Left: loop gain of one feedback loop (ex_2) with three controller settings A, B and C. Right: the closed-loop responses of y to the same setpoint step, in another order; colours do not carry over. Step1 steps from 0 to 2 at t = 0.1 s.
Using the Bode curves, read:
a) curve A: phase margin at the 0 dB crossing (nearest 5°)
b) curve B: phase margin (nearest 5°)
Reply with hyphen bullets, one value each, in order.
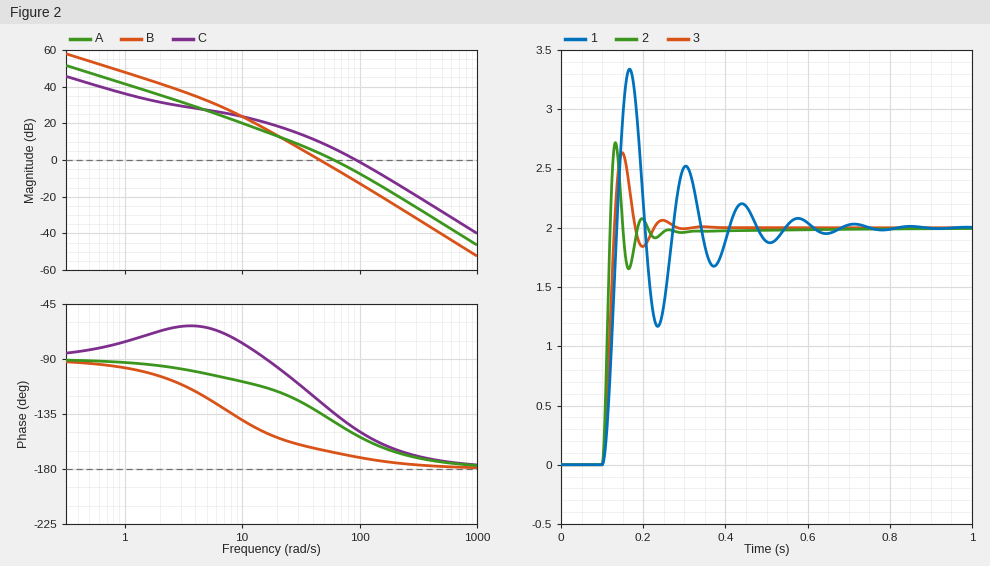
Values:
- 40°
- 15°
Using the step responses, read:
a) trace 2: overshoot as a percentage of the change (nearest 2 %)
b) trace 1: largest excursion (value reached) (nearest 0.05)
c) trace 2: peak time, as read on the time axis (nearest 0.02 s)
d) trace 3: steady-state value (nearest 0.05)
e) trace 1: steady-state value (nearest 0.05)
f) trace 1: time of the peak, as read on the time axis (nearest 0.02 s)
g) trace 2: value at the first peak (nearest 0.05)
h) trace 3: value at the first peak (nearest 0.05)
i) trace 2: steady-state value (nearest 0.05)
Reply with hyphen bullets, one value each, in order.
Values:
- 36 %
- 3.35
- 0.14 s
- 2.00
- 2.00
- 0.16 s
- 2.70
- 2.65
- 2.00
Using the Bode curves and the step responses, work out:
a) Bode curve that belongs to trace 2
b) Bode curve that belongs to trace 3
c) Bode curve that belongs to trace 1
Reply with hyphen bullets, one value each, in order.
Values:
- C
- A
- B
